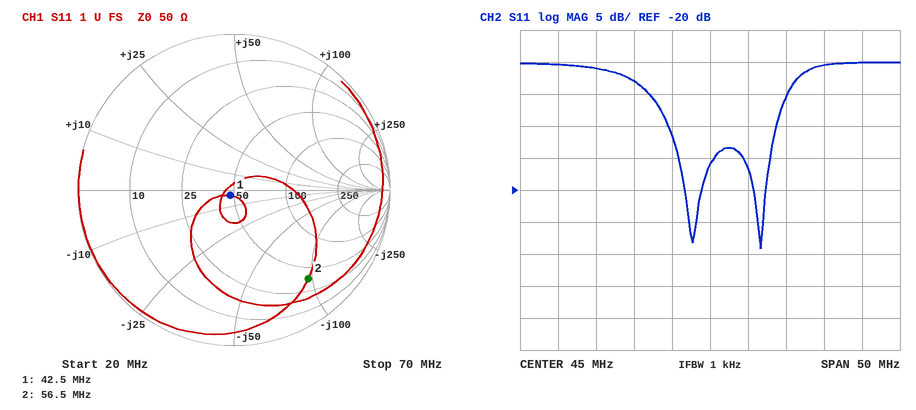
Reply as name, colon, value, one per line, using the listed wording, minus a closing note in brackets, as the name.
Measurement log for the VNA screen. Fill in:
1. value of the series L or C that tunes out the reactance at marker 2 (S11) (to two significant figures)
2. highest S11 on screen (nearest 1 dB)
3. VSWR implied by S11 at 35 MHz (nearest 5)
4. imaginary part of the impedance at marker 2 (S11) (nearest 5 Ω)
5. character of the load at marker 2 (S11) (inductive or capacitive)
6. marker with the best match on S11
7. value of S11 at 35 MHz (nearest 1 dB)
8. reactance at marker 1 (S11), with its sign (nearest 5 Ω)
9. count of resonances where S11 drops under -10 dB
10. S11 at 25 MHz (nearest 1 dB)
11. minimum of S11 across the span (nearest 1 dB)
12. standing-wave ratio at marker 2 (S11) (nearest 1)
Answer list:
value of the series L or C that tunes out the reactance at marker 2 (S11): 270 nH
highest S11 on screen: 0 dB
VSWR implied by S11 at 35 MHz: 5
imaginary part of the impedance at marker 2 (S11): -95 Ω
character of the load at marker 2 (S11): capacitive
marker with the best match on S11: marker 1
value of S11 at 35 MHz: -3 dB
reactance at marker 1 (S11), with its sign: -5 Ω
count of resonances where S11 drops under -10 dB: 2
S11 at 25 MHz: 0 dB
minimum of S11 across the span: -29 dB
standing-wave ratio at marker 2 (S11): 7
